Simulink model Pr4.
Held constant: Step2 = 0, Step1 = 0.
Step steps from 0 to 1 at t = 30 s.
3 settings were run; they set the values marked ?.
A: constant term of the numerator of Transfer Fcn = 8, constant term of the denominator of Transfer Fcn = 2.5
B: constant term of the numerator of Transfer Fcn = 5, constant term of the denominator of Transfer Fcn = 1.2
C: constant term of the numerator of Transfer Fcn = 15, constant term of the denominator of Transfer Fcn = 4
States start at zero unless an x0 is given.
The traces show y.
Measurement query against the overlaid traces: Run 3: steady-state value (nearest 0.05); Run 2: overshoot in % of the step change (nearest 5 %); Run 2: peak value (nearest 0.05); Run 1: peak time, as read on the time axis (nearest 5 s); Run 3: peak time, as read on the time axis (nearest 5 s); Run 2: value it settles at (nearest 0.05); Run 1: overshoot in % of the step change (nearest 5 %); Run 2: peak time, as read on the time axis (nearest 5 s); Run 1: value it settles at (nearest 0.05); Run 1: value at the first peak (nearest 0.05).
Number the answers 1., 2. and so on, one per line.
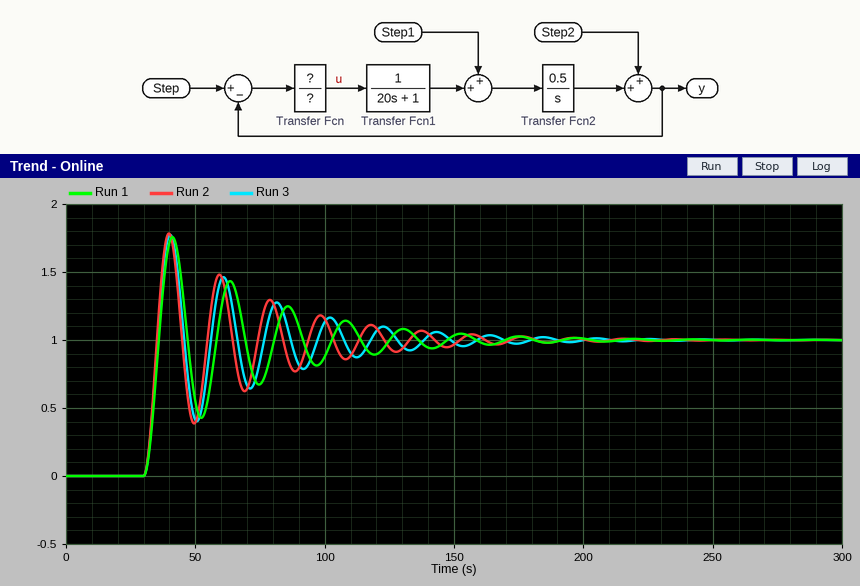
1. 1.00
2. 80 %
3. 1.80
4. 40 s
5. 40 s
6. 1.00
7. 75 %
8. 40 s
9. 1.00
10. 1.75
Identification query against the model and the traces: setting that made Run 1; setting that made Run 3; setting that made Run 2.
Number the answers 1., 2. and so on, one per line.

1. A
2. C
3. B
